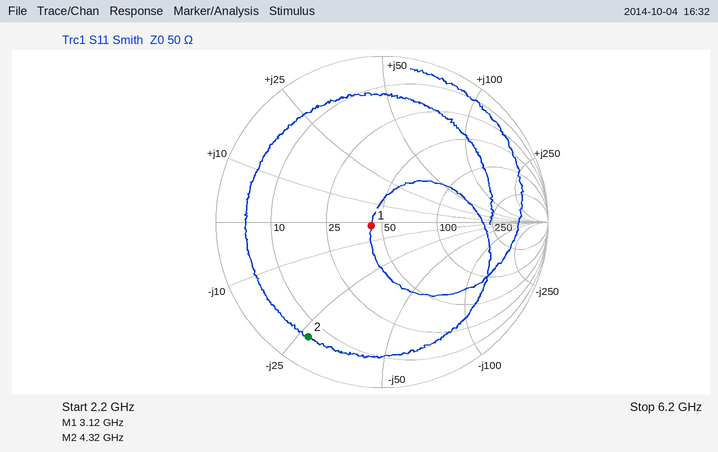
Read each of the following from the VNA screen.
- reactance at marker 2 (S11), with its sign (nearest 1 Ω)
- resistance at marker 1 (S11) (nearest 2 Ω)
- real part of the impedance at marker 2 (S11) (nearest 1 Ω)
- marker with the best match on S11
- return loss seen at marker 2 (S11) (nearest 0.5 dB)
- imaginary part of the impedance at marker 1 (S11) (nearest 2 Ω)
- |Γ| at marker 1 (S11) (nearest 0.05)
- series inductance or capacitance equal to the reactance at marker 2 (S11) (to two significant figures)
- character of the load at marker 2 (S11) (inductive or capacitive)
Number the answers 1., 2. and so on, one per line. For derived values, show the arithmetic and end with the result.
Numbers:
1. -27 Ω
2. 44 Ω
3. 6 Ω
4. marker 1
5. 1.5 dB
6. -2 Ω
7. 0.05
8. C = 1/(2π × 4.32 GHz × 27 Ω) ≈ 1.4 pF
9. capacitive
